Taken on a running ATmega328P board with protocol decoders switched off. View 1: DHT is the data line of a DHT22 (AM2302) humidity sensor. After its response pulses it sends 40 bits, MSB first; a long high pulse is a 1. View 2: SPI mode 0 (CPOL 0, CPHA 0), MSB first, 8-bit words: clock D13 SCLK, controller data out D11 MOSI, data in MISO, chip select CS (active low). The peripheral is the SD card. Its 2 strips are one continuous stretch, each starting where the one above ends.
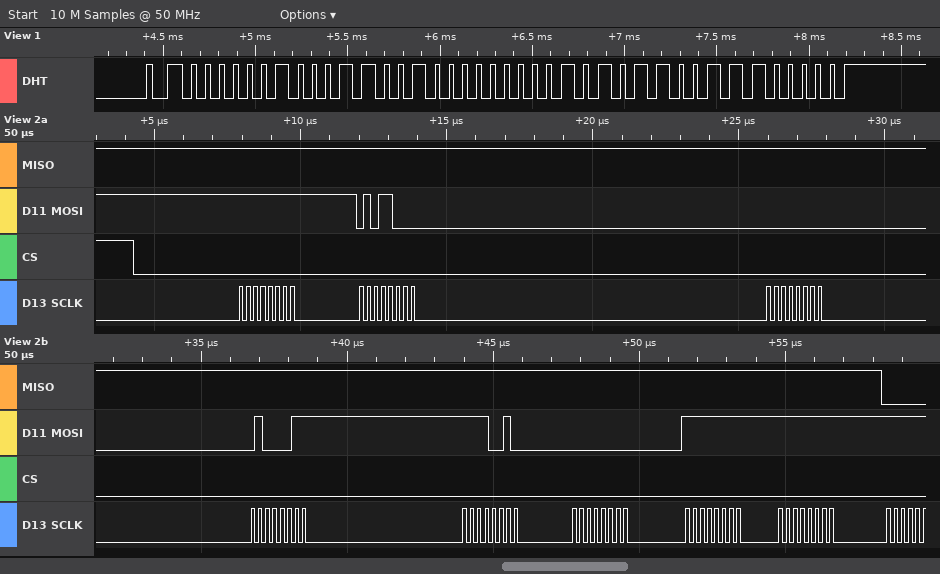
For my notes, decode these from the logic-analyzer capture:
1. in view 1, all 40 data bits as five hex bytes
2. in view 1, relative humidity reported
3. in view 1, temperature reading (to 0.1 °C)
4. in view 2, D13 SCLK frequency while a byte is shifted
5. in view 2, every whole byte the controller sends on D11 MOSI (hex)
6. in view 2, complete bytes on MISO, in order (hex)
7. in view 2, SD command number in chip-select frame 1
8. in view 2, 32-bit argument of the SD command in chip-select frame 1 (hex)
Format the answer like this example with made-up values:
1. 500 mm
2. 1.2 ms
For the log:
1. 02 32 00 AC E0
2. 56.2 %
3. 17.2 °C
4. 4 MHz
5. FF 58 00 43 F2 00 FF FF
6. FF FF FF FF FF FF FF FF
7. CMD24
8. 0x0043F200
